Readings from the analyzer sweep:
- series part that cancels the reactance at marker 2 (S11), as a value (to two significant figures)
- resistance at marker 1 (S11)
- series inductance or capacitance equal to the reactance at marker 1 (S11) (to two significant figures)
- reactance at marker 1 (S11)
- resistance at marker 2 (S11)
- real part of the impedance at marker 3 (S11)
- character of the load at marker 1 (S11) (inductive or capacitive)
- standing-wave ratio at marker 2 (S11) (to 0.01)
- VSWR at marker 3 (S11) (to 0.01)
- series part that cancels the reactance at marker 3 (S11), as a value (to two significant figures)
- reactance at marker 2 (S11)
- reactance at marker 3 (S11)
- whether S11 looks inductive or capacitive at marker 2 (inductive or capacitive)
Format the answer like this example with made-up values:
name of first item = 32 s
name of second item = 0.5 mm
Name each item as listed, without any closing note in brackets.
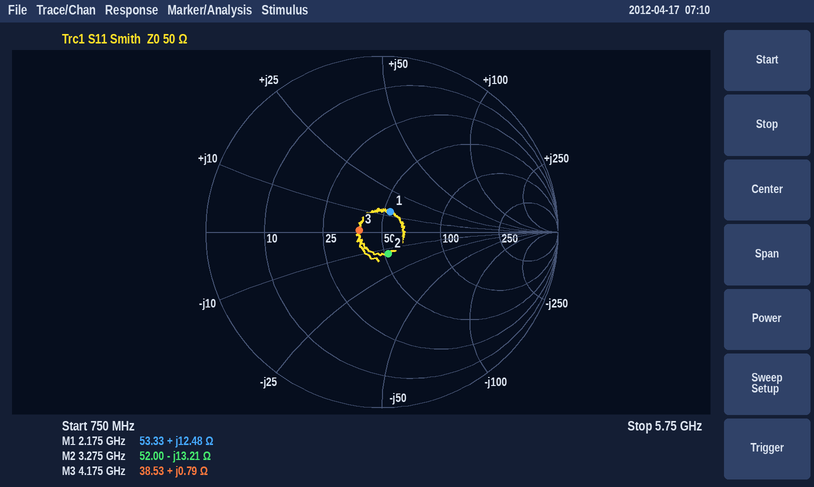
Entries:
series part that cancels the reactance at marker 2 (S11), as a value = 640 pH
resistance at marker 1 = 53.33 Ω
series inductance or capacitance equal to the reactance at marker 1 (S11) = 910 pH
reactance at marker 1 = +12.48 Ω
resistance at marker 2 = 52.00 Ω
real part of the impedance at marker 3 = 38.53 Ω
character of the load at marker 1 (S11) = inductive
standing-wave ratio at marker 2 (S11) = 1.30
VSWR at marker 3 (S11) = 1.30
series part that cancels the reactance at marker 3 (S11), as a value = 48 pF
reactance at marker 2 = -13.21 Ω
reactance at marker 3 = +0.79 Ω
whether S11 looks inductive or capacitive at marker 2 = capacitive
